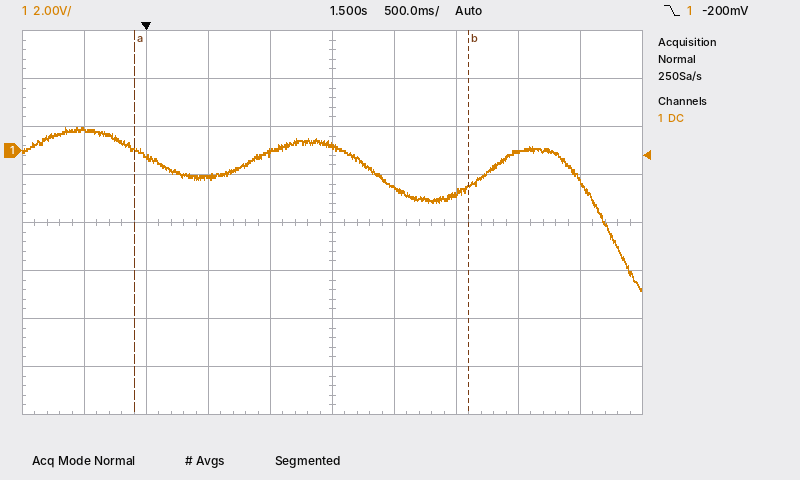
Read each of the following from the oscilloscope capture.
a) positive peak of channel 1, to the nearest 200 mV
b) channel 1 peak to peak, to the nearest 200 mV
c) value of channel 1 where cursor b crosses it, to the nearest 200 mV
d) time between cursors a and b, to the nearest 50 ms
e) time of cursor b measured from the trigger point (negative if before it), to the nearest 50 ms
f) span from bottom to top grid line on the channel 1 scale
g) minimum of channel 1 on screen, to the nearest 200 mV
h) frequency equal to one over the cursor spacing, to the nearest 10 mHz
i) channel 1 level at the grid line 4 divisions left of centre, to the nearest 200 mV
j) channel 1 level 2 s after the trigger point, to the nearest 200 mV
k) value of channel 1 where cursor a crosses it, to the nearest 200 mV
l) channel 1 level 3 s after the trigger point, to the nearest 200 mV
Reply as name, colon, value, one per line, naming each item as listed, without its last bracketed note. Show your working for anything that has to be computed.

positive peak of channel 1, to the nearest 200 mV: 1.0 V
channel 1 peak to peak, to the nearest 200 mV: 1.0 V − (-5.8 V) = 6.8 V
value of channel 1 where cursor b crosses it, to the nearest 200 mV: -1.6 V
time between cursors a and b, to the nearest 50 ms: 2.70 s
time of cursor b measured from the trigger point (negative if before it), to the nearest 50 ms: +2.60 s
span from bottom to top grid line on the channel 1 scale: 16 V
minimum of channel 1 on screen, to the nearest 200 mV: -5.8 V
frequency equal to one over the cursor spacing, to the nearest 10 mHz: 1 / 2.70 s ≈ 370 mHz
channel 1 level at the grid line 4 divisions left of centre, to the nearest 200 mV: 800 mV
channel 1 level 2 s after the trigger point, to the nearest 200 mV: -1.6 V
value of channel 1 where cursor a crosses it, to the nearest 200 mV: 0.0 V
channel 1 level 3 s after the trigger point, to the nearest 200 mV: 0.0 V
